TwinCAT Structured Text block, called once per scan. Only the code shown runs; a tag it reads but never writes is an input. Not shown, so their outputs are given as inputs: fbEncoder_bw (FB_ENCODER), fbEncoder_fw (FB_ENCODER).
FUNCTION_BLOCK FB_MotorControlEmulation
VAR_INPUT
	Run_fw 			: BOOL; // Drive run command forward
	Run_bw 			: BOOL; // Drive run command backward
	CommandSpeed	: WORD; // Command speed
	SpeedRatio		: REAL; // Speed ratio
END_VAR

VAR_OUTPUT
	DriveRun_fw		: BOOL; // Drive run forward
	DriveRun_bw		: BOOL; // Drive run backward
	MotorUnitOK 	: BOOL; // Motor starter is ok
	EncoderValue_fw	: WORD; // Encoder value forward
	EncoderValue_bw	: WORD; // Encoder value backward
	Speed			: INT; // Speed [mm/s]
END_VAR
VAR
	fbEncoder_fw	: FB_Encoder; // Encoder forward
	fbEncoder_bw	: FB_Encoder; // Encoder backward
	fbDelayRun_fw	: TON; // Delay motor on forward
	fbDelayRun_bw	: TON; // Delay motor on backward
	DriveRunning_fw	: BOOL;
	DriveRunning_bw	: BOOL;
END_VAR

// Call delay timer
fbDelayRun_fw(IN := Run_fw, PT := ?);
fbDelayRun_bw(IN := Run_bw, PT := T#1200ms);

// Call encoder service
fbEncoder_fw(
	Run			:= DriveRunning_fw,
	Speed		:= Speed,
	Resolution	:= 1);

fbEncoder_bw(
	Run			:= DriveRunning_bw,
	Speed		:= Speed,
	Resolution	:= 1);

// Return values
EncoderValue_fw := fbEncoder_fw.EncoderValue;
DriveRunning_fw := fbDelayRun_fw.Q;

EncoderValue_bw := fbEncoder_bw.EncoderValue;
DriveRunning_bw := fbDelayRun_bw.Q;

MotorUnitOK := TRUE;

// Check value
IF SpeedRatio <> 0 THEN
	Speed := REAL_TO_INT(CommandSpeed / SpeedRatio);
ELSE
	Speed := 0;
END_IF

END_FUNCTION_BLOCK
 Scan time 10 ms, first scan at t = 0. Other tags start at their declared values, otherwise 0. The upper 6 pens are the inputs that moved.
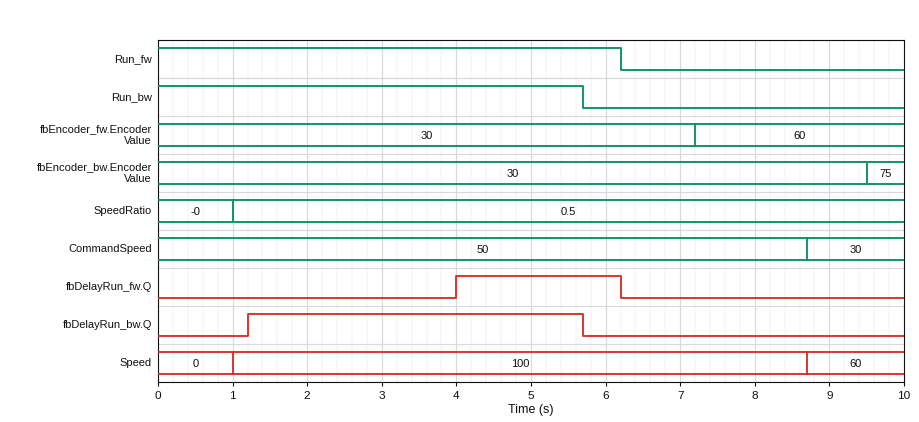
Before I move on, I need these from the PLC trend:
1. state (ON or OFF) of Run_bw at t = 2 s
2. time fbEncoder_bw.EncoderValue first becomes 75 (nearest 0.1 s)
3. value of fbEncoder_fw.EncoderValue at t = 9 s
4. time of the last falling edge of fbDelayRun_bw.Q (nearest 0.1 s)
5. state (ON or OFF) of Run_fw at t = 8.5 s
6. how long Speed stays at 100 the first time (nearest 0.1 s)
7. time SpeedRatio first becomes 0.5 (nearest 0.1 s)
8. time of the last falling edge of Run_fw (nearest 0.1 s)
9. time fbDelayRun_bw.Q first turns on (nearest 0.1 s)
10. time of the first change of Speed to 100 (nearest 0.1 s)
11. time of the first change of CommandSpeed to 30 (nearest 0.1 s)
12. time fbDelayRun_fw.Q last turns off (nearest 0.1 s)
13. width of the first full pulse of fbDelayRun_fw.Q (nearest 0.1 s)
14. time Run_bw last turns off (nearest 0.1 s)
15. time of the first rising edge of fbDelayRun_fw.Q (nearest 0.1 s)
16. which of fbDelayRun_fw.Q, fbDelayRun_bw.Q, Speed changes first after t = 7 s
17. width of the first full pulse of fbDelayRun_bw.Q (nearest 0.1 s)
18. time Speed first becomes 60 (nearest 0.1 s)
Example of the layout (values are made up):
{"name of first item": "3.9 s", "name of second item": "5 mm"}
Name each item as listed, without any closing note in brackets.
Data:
{"state (ON or OFF) of Run_bw at t = 2 s": "ON", "time fbEncoder_bw.EncoderValue first becomes 75": "9.5 s", "value of fbEncoder_fw.EncoderValue at t = 9 s": "60", "time of the last falling edge of fbDelayRun_bw.Q": "5.7 s", "state (ON or OFF) of Run_fw at t = 8.5 s": "OFF", "how long Speed stays at 100 the first time": "7.7 s", "time SpeedRatio first becomes 0.5": "1.0 s", "time of the last falling edge of Run_fw": "6.2 s", "time fbDelayRun_bw.Q first turns on": "1.2 s", "time of the first change of Speed to 100": "1.0 s", "time of the first change of CommandSpeed to 30": "8.7 s", "time fbDelayRun_fw.Q last turns off": "6.2 s", "width of the first full pulse of fbDelayRun_fw.Q": "2.2 s", "time Run_bw last turns off": "5.7 s", "time of the first rising edge of fbDelayRun_fw.Q": "4.0 s", "which of fbDelayRun_fw.Q, fbDelayRun_bw.Q, Speed changes first after t = 7 s": "Speed", "width of the first full pulse of fbDelayRun_bw.Q": "4.5 s", "time Speed first becomes 60": "8.7 s"}
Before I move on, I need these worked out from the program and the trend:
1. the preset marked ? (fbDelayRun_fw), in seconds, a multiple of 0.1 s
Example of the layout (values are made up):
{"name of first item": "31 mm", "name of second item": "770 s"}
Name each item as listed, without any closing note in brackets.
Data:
{"the preset marked ? (fbDelayRun_fw), in seconds, a multiple of 0.1 s": "4.0 s"}
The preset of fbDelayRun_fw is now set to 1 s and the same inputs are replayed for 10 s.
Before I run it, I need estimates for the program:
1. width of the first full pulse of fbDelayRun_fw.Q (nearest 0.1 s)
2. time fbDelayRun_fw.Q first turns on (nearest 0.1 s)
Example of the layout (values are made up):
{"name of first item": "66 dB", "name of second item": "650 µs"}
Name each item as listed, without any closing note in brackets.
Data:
{"width of the first full pulse of fbDelayRun_fw.Q": "5.2 s", "time fbDelayRun_fw.Q first turns on": "1.0 s"}
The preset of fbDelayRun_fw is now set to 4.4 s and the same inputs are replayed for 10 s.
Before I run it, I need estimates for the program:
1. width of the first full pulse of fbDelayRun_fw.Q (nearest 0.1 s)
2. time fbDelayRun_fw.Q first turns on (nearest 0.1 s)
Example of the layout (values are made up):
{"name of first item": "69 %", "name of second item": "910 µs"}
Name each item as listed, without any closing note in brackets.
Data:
{"width of the first full pulse of fbDelayRun_fw.Q": "1.8 s", "time fbDelayRun_fw.Q first turns on": "4.4 s"}
